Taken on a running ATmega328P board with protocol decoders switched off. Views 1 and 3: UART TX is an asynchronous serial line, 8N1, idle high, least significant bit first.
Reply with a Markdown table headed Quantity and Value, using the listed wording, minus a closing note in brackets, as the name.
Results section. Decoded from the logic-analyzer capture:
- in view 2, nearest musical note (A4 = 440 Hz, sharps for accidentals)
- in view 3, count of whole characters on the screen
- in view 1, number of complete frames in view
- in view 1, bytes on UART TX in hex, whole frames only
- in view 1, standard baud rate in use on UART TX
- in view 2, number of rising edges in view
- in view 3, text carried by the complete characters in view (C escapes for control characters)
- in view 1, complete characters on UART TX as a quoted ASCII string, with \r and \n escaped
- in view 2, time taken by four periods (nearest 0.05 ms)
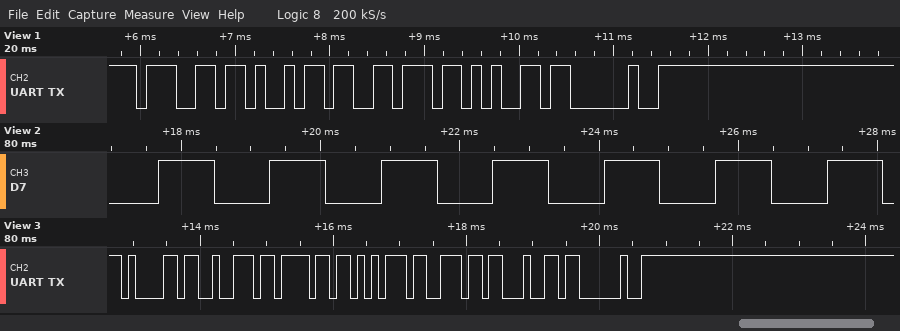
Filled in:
| Quantity | Value |
|---|---|
| in view 2, nearest musical note | D#5 |
| in view 3, count of whole characters on the screen | 7 |
| in view 1, number of complete frames in view | 5 |
| in view 1, bytes on UART TX in hex, whole frames only | 67 69 76 65 20 |
| in view 1, standard baud rate in use on UART TX | 9600 baud |
| in view 2, number of rising edges in view | 7 |
| in view 3, text carried by the complete characters in view | "around " |
| in view 1, complete characters on UART TX as a quoted ASCII string, with \r and \n escaped | "give " |
| in view 2, time taken by four periods | 6.40 ms |
